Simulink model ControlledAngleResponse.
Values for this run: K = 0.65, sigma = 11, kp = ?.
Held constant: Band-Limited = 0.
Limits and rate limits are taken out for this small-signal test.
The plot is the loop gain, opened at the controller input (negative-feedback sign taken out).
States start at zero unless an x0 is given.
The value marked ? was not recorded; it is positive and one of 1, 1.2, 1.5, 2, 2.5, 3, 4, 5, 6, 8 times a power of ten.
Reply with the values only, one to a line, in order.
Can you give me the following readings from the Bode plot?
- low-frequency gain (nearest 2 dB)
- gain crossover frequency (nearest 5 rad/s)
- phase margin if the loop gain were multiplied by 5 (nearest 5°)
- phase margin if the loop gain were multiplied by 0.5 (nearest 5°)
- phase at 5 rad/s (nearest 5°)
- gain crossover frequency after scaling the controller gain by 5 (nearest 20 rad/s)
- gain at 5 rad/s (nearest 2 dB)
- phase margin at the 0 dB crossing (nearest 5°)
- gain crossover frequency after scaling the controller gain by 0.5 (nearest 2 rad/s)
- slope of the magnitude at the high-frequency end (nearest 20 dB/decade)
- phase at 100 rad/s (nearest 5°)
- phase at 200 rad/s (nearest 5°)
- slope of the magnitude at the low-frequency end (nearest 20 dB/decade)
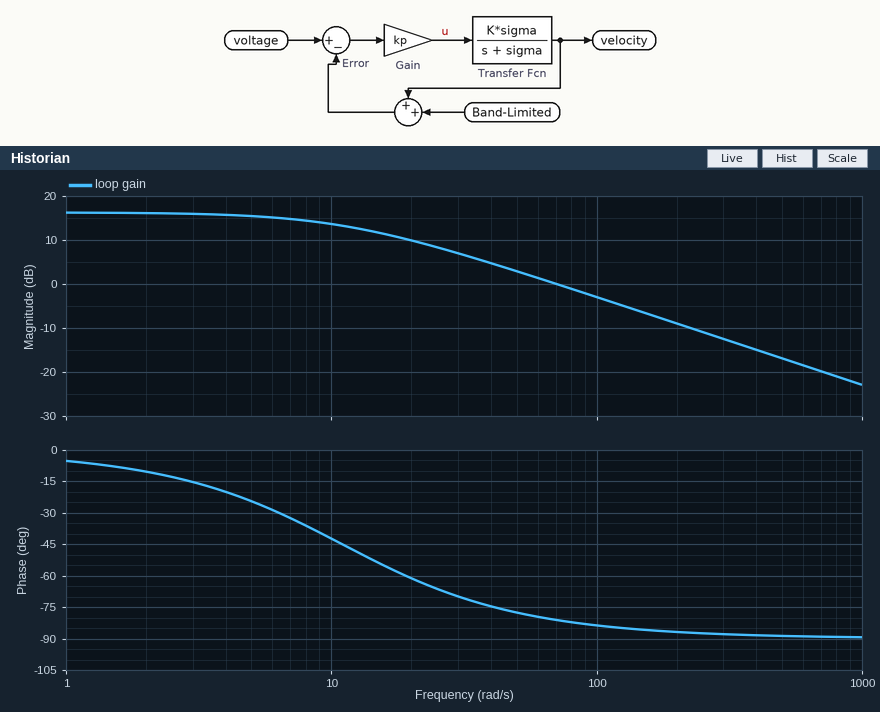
16 dB
70 rad/s
90°
110°
-25°
360 rad/s
16 dB
100°
34 rad/s
-20 dB/decade
-85°
-85°
0 dB/decade
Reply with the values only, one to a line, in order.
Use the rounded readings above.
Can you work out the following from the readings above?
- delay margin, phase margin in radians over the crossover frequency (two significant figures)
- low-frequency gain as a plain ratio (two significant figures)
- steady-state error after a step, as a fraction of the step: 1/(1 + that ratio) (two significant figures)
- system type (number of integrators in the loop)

0.025 s
6.3
0.14
0
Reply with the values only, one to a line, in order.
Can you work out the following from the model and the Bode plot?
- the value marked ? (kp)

10
